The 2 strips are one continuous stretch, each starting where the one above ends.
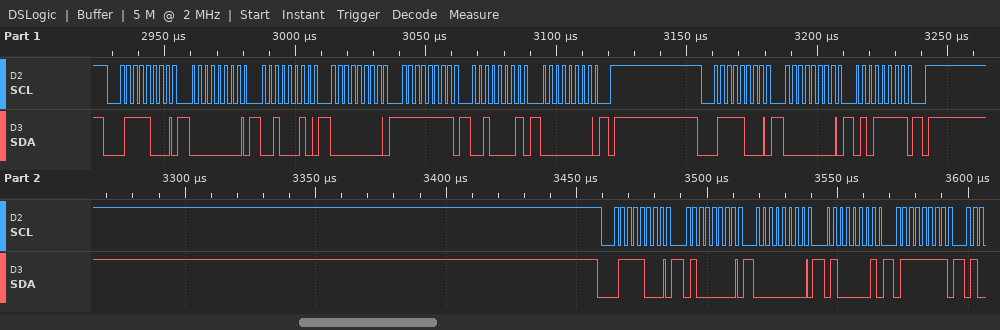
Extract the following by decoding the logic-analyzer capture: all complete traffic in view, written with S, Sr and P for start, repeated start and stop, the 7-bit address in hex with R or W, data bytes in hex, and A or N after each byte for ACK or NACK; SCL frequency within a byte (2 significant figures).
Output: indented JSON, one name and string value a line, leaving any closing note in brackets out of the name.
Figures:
{
  "all complete traffic in view, written with S, Sr and P for start, repeated start and stop, the 7-bit address in hex with R or W, data bytes in hex, and A or N after each byte for ACK or NACK": "S 3CW A 00 A 22 A 00 A FF A 21 A 00 A P S 3CW A 00 A 5F A P S 3CW A 40 A 00 A 41 A 7F A",
  "SCL frequency within a byte": "400 kHz"
}
